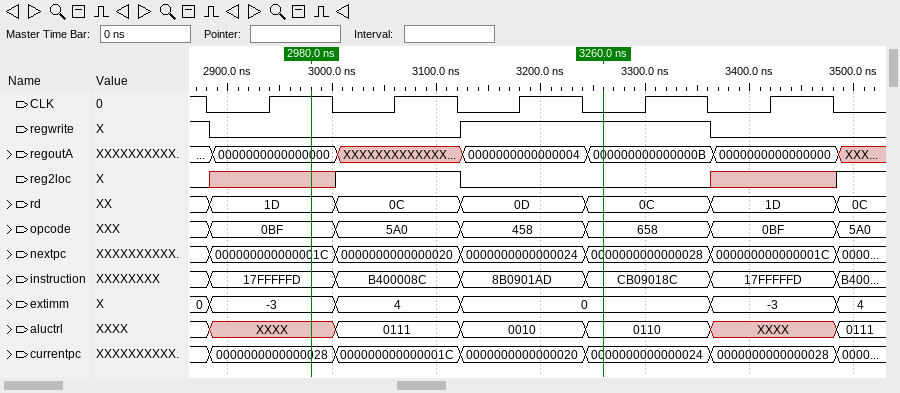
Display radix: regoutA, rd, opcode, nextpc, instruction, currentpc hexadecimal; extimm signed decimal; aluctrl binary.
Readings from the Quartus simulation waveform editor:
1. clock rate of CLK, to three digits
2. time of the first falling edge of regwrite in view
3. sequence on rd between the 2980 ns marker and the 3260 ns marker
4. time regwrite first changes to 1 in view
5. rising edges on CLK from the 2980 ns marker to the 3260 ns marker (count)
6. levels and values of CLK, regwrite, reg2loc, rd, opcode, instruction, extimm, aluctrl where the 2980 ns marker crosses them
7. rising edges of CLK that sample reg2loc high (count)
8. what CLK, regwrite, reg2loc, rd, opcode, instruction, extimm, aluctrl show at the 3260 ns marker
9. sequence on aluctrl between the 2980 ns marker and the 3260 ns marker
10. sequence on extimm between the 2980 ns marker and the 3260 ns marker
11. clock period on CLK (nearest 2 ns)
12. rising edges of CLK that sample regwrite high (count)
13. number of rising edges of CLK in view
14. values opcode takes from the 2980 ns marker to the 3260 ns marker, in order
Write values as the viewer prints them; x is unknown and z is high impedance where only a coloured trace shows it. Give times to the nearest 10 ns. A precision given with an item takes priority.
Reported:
8.33 MHz
2880 ns
1D, 0C, 0D, 0C
3120 ns
2
CLK=1, regwrite=0, reg2loc=x, rd=1D, opcode=0BF, instruction=17FFFFFD, extimm=-3, aluctrl=XXXX
1
CLK=0, regwrite=1, reg2loc=0, rd=0C, opcode=658, instruction=CB09018C, extimm=0, aluctrl=0110
XXXX, 0111, 0010, 0110
-3, 4, 0
120 ns
2
5
0BF, 5A0, 458, 658
